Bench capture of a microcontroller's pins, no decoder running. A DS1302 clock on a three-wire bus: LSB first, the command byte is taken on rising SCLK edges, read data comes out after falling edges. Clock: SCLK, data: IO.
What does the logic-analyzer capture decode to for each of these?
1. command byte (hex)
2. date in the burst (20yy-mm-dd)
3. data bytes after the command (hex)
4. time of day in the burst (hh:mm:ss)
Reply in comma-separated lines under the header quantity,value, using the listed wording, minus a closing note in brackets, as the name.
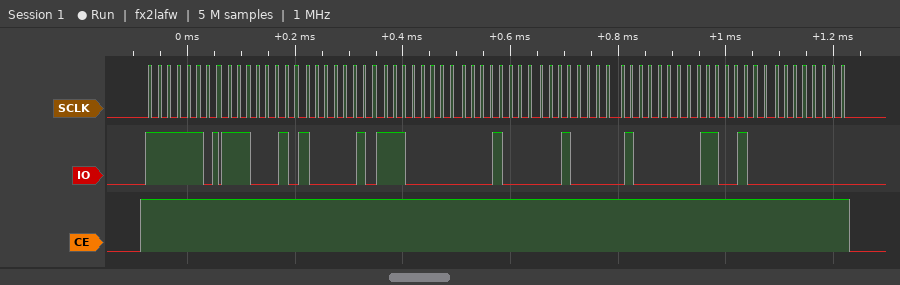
quantity,value
command byte,0xBF
date in the burst,2026-08-10
data bytes after the command,47 41 07 10 08 02 26 00
time of day in the burst,07:41:47
